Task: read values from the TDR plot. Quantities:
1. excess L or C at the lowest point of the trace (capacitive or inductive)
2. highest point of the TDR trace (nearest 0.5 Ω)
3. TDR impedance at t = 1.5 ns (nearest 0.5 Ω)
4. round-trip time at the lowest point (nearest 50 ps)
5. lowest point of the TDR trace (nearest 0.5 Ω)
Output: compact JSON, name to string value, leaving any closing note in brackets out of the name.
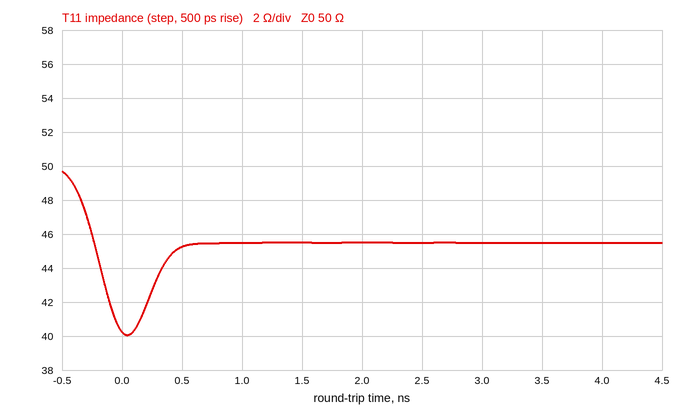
{"excess L or C at the lowest point of the trace": "capacitive", "highest point of the TDR trace": "49.5 Ω", "TDR impedance at t = 1.5 ns": "45.5 Ω", "round-trip time at the lowest point": "50 ps", "lowest point of the TDR trace": "40.0 Ω"}
